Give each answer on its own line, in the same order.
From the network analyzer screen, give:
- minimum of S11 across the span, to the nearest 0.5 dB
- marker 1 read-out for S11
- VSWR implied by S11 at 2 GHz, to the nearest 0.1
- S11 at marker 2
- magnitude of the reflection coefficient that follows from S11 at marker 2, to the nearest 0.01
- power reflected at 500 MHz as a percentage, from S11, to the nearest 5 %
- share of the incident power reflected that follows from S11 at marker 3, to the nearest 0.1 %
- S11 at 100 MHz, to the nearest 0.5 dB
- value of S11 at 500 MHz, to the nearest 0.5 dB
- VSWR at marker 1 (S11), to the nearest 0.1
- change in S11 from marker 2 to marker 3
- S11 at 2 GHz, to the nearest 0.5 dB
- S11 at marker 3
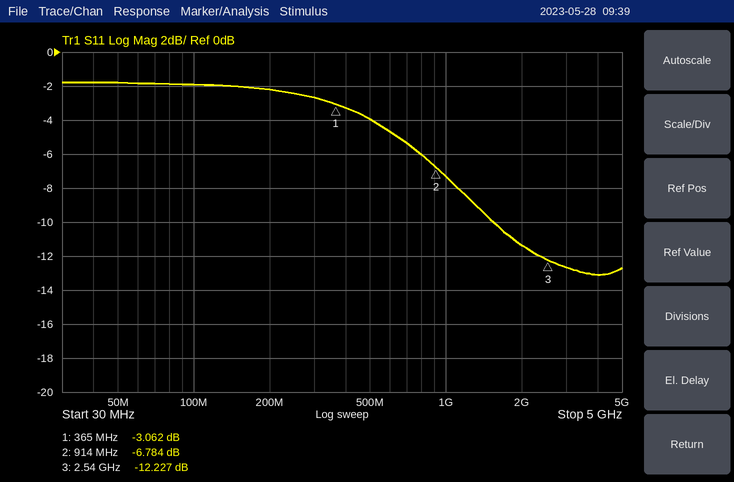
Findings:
-13.0 dB
-3.062 dB
1.7
-6.784 dB
0.46
40 %
6.0 %
-2.0 dB
-4.0 dB
5.7
-5.443 dB
-11.5 dB
-12.227 dB
